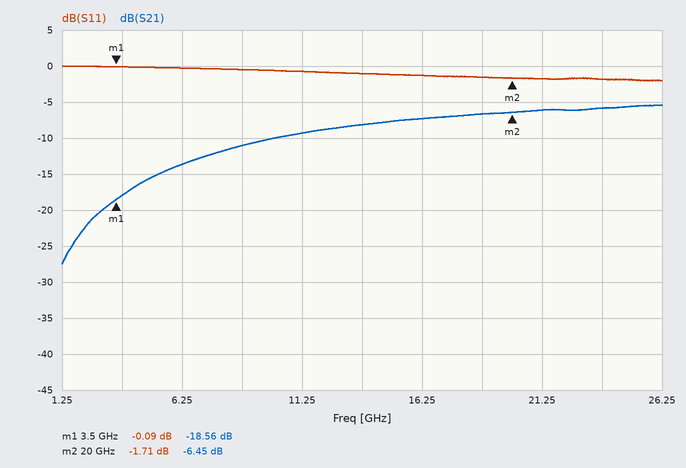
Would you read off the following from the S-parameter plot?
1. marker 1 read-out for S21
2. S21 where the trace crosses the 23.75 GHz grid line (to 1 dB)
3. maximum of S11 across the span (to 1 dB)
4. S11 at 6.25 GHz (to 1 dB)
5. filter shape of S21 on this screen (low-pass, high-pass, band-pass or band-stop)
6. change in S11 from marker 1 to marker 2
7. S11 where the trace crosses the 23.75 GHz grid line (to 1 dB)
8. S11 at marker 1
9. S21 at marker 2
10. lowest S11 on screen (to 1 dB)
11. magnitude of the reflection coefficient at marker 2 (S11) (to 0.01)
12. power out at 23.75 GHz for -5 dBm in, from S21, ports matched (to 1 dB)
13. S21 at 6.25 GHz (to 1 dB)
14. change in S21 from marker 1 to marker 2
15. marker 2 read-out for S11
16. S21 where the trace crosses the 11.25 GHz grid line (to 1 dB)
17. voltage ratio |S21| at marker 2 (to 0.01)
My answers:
-18.56 dB
-6 dB
0 dB
0 dB
high-pass
-1.62 dB
-2 dB
-0.09 dB
-6.45 dB
-2 dB
0.82
-11 dBm
-14 dB
12.11 dB
-1.71 dB
-9 dB
0.48
